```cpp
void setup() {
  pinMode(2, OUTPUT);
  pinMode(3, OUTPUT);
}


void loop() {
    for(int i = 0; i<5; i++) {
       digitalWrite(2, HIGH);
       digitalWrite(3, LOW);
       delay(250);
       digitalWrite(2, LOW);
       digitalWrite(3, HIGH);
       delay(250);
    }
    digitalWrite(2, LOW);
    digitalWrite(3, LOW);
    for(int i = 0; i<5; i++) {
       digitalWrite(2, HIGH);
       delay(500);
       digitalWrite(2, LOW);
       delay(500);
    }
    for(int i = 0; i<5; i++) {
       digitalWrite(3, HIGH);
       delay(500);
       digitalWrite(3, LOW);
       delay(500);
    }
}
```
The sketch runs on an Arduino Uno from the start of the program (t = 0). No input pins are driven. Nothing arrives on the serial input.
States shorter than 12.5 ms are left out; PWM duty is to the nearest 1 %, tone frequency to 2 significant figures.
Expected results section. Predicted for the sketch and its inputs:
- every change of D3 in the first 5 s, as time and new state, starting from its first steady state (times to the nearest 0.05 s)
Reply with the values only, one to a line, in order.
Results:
0 s low; 0.25 s high; 0.5 s low; 0.75 s high; 1 s low; 1.25 s high; 1.5 s low; 1.75 s high; 2 s low; 2.25 s high; 2.5 s low
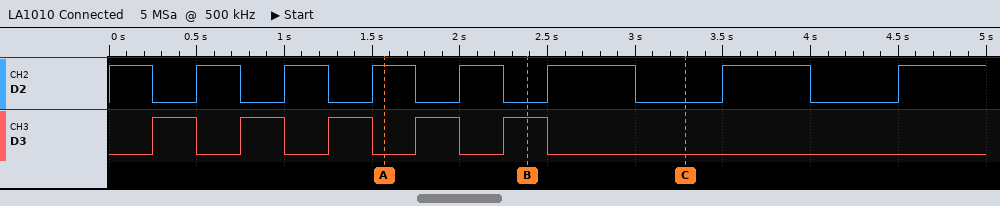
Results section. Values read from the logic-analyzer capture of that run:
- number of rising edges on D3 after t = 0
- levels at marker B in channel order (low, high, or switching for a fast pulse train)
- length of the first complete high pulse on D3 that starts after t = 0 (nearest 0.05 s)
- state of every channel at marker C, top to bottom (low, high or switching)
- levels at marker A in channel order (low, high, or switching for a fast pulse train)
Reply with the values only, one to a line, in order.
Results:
5
D2 low, D3 high
0.25 s
D2 low, D3 low
D2 high, D3 low
